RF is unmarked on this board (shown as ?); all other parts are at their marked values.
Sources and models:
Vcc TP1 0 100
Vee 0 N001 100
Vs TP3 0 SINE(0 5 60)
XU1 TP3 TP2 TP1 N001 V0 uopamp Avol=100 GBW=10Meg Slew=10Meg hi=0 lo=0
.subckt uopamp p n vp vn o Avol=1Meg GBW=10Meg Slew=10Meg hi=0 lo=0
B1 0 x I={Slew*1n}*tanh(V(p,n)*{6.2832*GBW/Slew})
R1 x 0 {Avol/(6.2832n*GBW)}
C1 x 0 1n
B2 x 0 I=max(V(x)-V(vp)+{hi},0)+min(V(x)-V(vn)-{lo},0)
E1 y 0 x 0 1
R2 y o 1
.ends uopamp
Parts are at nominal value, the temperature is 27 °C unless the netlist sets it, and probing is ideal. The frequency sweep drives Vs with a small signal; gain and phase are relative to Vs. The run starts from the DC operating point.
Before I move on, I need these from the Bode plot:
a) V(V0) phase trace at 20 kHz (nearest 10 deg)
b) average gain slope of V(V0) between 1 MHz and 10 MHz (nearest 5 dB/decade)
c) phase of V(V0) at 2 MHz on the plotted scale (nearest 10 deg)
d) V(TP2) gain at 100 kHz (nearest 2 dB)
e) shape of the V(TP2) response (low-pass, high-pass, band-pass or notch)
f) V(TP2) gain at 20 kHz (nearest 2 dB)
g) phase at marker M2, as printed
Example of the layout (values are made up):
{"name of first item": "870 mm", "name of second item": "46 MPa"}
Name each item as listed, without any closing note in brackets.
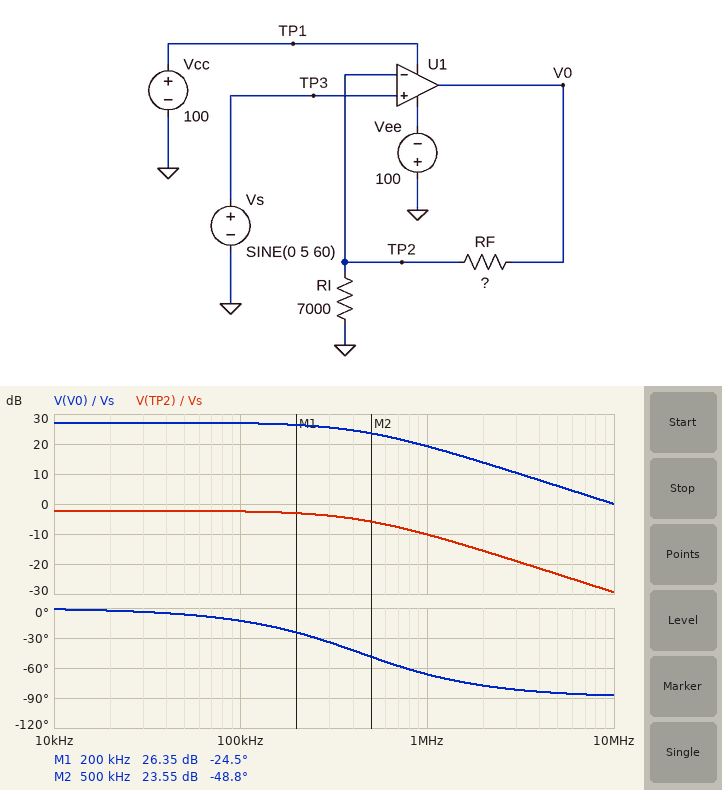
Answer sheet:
{"V(V0) phase trace at 20 kHz": "0 deg", "average gain slope of V(V0) between 1 MHz and 10 MHz": "-20 dB/decade", "phase of V(V0) at 2 MHz on the plotted scale": "-80 deg", "V(TP2) gain at 100 kHz": "-2 dB", "shape of the V(TP2) response": "low-pass", "V(TP2) gain at 20 kHz": "-2 dB", "phase at marker M2, as printed": "-48.8 deg"}
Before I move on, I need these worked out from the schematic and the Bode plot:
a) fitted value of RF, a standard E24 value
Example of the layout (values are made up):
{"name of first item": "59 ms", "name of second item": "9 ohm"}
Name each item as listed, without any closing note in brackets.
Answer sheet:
{"fitted value of RF, a standard E24 value": "200 kΩ"}
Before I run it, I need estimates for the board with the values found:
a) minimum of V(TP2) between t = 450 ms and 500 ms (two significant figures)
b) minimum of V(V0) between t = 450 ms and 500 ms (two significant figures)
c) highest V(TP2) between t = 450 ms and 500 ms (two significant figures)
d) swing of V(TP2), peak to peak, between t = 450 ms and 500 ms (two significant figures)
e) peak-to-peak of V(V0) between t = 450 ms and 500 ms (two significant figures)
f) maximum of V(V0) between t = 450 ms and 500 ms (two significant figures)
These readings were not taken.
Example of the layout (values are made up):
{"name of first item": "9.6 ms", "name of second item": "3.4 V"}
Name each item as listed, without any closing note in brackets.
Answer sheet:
{"minimum of V(TP2) between t = 450 ms and 500 ms": "-540 mV", "minimum of V(V0) between t = 450 ms and 500 ms": "-16 V", "highest V(TP2) between t = 450 ms and 500 ms": "540 mV", "swing of V(TP2), peak to peak, between t = 450 ms and 500 ms": "1.1 V", "peak-to-peak of V(V0) between t = 450 ms and 500 ms": "32 V", "maximum of V(V0) between t = 450 ms and 500 ms": "16 V"}
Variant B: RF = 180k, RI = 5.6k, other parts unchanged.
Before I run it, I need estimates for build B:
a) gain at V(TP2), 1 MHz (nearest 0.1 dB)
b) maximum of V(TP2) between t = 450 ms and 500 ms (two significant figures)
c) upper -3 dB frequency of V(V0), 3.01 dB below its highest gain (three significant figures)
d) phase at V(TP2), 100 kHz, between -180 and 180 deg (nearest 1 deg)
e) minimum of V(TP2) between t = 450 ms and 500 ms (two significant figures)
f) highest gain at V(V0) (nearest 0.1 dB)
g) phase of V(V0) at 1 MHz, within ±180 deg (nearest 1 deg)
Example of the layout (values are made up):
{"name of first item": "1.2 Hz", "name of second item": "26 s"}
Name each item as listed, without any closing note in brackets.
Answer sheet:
{"gain at V(TP2), 1 MHz": "-11.1 dB", "maximum of V(TP2) between t = 450 ms and 500 ms": "480 mV", "upper -3 dB frequency of V(V0), 3.01 dB below its highest gain": "402 kHz", "phase at V(TP2), 100 kHz, between -180 and 180 deg": "-14 deg", "minimum of V(TP2) between t = 450 ms and 500 ms": "-480 mV", "highest gain at V(V0)": "27.9 dB", "phase of V(V0) at 1 MHz, within ±180 deg": "-68 deg"}
